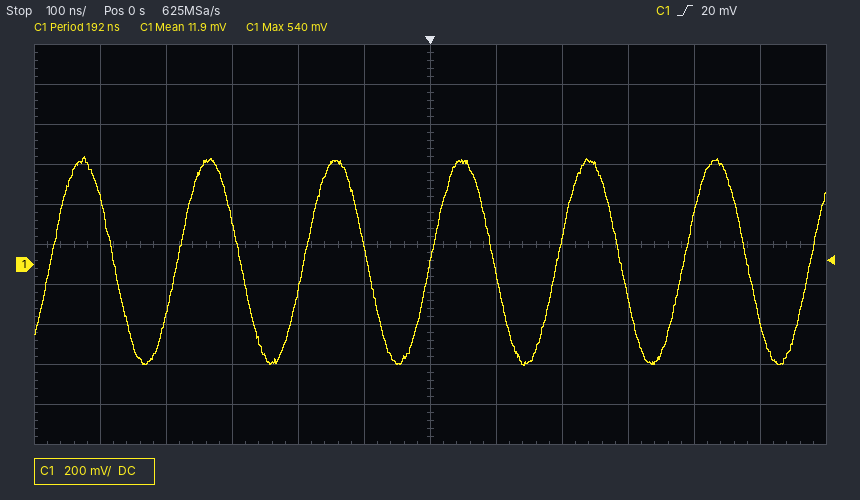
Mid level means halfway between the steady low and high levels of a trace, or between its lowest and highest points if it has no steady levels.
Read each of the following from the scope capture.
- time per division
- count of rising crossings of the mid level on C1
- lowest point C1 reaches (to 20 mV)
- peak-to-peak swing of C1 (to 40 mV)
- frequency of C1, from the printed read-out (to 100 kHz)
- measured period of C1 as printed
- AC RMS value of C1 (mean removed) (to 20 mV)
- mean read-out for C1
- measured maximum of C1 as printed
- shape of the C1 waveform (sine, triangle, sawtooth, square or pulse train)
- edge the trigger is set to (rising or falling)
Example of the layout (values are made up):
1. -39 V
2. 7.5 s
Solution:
1. 100 ns
2. 7
3. -500 mV
4. 1.04 V
5. 5.2 MHz
6. 192 ns
7. 360 mV
8. 11.9 mV
9. 540 mV
10. sine
11. rising
